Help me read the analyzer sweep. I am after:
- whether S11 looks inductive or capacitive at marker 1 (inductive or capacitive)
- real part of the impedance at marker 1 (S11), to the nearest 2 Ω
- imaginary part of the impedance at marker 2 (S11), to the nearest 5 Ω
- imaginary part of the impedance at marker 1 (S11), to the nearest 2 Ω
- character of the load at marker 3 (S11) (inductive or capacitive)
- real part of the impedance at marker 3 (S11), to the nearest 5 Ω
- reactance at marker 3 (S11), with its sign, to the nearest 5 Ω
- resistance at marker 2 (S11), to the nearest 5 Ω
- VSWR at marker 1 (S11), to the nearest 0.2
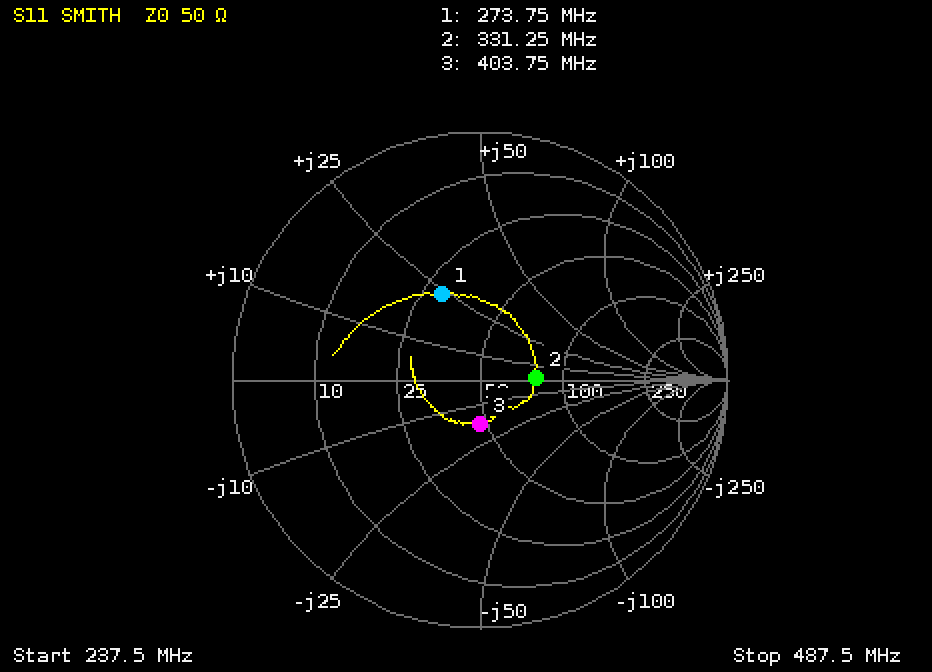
inductive
30 Ω
0 Ω
+24 Ω
capacitive
45 Ω
-15 Ω
80 Ω
2.2
